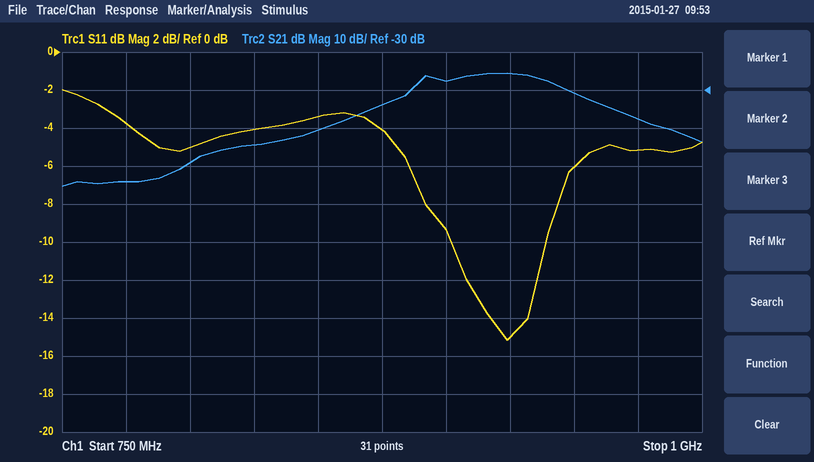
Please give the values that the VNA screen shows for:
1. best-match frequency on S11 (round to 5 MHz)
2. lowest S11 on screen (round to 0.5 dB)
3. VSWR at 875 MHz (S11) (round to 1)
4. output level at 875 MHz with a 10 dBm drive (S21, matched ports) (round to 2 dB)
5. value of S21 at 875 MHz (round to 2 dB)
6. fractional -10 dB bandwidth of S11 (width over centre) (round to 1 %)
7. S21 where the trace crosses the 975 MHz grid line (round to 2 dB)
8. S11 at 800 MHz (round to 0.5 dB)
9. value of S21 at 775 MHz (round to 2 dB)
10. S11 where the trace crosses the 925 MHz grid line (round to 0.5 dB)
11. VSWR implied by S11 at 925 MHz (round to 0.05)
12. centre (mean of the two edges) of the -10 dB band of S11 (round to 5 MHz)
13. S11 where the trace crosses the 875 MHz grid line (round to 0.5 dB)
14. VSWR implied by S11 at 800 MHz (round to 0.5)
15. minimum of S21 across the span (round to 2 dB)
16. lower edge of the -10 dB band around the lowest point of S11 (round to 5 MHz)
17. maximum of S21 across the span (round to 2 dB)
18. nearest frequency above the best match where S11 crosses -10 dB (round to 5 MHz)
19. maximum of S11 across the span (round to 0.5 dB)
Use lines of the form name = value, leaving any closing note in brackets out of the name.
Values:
best-match frequency on S11 = 925 MHz
lowest S11 on screen = -15.0 dB
VSWR at 875 MHz (S11) = 4
output level at 875 MHz with a 10 dBm drive (S21, matched ports) = -24 dBm
value of S21 at 875 MHz = -34 dB
fractional -10 dB bandwidth of S11 (width over centre) = 4 %
S21 where the trace crosses the 975 MHz grid line = -38 dB
S11 at 800 MHz = -5.0 dB
value of S21 at 775 MHz = -54 dB
S11 where the trace crosses the 925 MHz grid line = -15.0 dB
VSWR implied by S11 at 925 MHz = 1.45
centre (mean of the two edges) of the -10 dB band of S11 = 920 MHz
S11 where the trace crosses the 875 MHz grid line = -4.0 dB
VSWR implied by S11 at 800 MHz = 3.5
minimum of S21 across the span = -56 dB
lower edge of the -10 dB band around the lowest point of S11 = 900 MHz
maximum of S21 across the span = -26 dB
nearest frequency above the best match where S11 crosses -10 dB = 940 MHz
maximum of S11 across the span = -2.0 dB
